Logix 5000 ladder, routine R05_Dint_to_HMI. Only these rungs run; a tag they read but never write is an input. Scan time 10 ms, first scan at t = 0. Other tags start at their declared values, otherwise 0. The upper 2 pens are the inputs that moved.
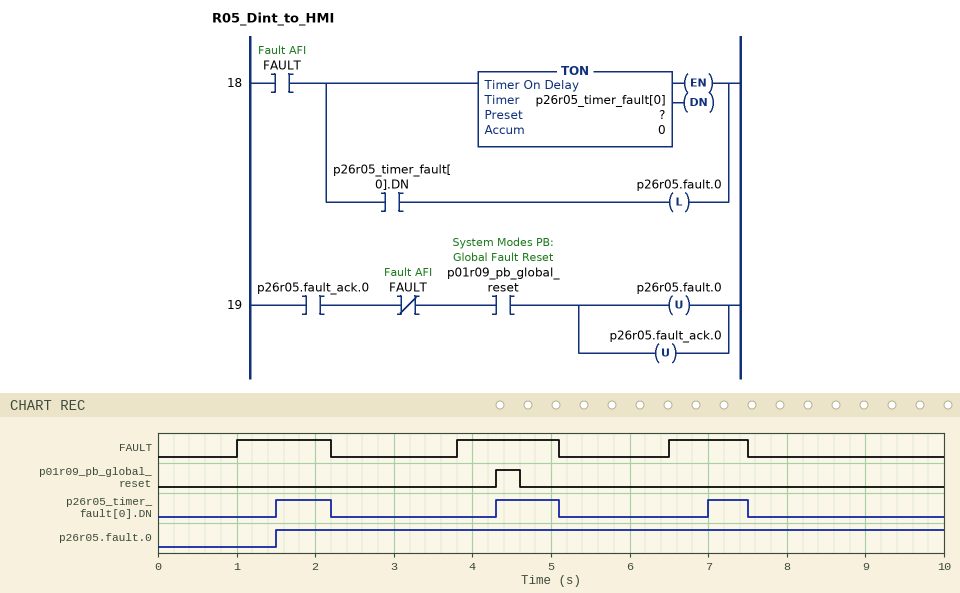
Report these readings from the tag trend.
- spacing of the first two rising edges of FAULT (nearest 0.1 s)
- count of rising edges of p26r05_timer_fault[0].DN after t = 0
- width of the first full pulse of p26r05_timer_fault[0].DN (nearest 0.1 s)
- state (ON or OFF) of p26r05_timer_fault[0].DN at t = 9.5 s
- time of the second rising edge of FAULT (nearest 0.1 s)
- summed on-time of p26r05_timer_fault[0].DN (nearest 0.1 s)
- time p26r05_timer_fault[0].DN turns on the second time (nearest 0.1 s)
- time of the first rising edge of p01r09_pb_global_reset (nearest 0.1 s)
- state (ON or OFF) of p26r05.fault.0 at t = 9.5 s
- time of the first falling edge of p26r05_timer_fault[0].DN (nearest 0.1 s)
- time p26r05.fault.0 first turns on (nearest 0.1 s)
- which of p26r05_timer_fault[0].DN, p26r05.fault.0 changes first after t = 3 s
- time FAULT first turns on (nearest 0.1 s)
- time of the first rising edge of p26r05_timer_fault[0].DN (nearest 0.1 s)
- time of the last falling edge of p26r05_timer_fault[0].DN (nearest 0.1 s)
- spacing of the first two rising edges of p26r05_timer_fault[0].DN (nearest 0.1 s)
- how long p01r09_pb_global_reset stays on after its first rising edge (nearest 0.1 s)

2.8 s
3
0.7 s
OFF
3.8 s
2.0 s
4.3 s
4.3 s
ON
2.2 s
1.5 s
p26r05_timer_fault[0].DN
1.0 s
1.5 s
7.5 s
2.8 s
0.3 s
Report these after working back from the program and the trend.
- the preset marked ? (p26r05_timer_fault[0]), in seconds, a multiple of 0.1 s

0.5 s
